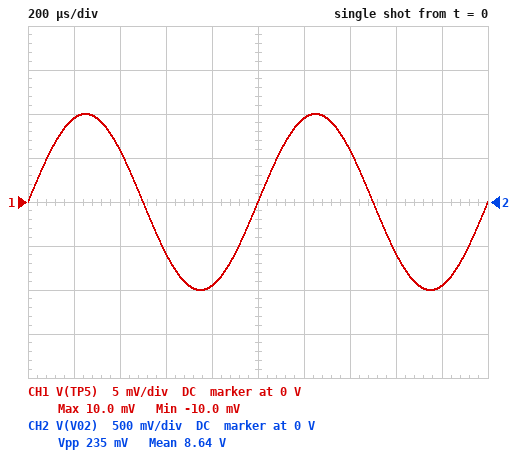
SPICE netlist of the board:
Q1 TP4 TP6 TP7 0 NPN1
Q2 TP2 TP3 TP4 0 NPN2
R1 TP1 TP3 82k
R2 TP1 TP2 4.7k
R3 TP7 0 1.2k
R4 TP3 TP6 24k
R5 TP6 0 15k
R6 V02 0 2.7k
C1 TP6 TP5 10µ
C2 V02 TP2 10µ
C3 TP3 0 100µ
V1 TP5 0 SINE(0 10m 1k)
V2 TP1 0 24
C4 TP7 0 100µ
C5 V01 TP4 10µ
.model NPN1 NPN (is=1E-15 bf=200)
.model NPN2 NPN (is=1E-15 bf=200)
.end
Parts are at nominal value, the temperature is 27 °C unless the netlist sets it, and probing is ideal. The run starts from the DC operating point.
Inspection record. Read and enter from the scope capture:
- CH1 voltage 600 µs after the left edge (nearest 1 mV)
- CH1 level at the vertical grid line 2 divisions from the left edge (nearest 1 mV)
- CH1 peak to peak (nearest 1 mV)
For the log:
-6 mV
6 mV
20 mV
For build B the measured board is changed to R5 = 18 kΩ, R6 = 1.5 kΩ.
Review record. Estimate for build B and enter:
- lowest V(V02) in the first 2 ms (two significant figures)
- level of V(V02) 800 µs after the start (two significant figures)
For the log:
5.6 V
5.7 V
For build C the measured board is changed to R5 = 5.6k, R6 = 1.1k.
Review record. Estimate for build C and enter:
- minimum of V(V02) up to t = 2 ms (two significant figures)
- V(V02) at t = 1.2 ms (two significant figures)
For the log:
4.4 V
4.5 V
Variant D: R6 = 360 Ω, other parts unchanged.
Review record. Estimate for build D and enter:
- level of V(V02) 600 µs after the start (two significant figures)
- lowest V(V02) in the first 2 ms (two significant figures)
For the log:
1.7 V
1.6 V
